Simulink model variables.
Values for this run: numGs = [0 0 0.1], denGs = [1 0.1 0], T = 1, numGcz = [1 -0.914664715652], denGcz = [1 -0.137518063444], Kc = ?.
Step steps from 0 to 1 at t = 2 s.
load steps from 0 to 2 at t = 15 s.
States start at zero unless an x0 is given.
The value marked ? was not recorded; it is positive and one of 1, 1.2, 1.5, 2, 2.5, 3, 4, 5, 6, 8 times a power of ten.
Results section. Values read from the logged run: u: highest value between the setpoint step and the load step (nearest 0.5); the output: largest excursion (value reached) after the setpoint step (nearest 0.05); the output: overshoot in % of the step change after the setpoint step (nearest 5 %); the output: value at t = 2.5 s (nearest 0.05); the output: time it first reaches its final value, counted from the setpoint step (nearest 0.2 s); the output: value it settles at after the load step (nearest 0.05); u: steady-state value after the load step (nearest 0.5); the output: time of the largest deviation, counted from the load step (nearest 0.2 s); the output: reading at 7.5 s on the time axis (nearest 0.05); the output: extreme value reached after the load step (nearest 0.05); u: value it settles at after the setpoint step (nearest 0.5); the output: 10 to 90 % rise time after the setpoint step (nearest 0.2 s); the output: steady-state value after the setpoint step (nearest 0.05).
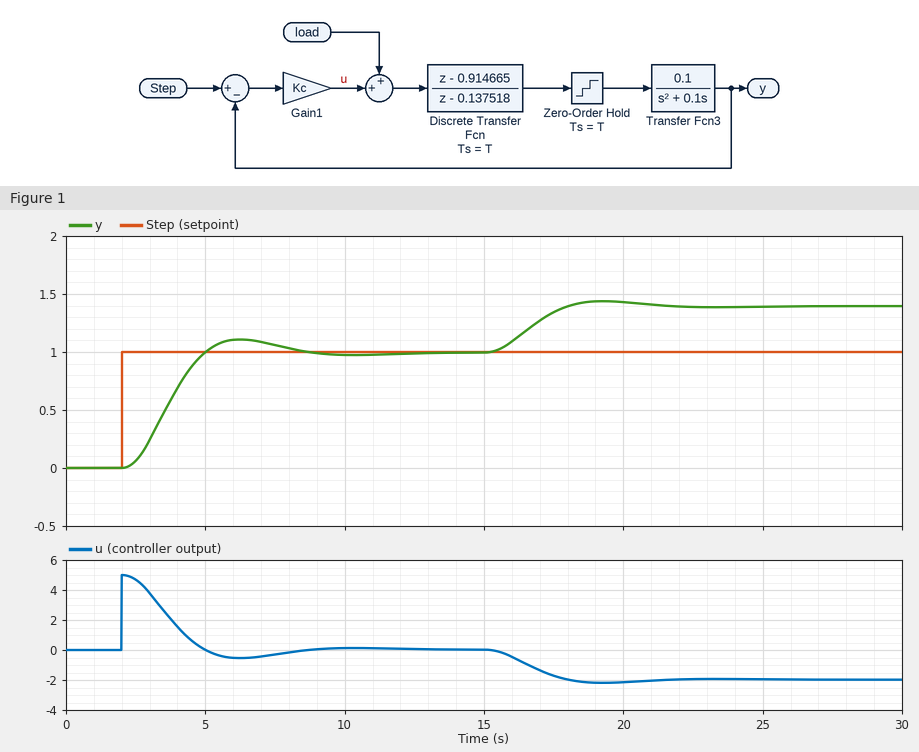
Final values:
5.0
1.10
10 %
0.05
3.0 s
1.40
-2.0
4.2 s
1.05
1.45
0.0
2.0 s
1.00
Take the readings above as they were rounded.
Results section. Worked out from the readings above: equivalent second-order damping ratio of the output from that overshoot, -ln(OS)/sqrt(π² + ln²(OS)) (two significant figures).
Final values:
0.59
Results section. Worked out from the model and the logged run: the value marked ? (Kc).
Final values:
5
